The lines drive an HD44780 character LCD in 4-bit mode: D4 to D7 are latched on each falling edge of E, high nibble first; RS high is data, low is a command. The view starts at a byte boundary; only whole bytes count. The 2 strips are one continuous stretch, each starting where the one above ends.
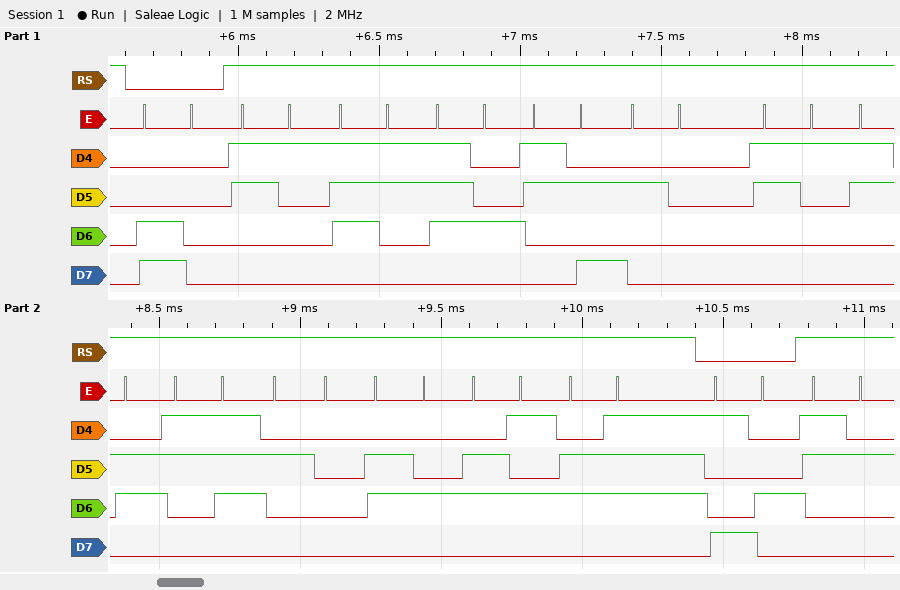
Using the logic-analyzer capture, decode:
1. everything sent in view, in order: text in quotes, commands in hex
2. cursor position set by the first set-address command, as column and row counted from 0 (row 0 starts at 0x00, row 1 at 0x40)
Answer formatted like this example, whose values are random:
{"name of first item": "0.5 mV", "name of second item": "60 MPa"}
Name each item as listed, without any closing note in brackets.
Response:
{"everything sent in view, in order: text in quotes, commands in hex": "0xC0 \"1st: 167 deg\" 0x94 \"2\"", "cursor position set by the first set-address command, as column and row counted from 0": "column 0, row 1"}
